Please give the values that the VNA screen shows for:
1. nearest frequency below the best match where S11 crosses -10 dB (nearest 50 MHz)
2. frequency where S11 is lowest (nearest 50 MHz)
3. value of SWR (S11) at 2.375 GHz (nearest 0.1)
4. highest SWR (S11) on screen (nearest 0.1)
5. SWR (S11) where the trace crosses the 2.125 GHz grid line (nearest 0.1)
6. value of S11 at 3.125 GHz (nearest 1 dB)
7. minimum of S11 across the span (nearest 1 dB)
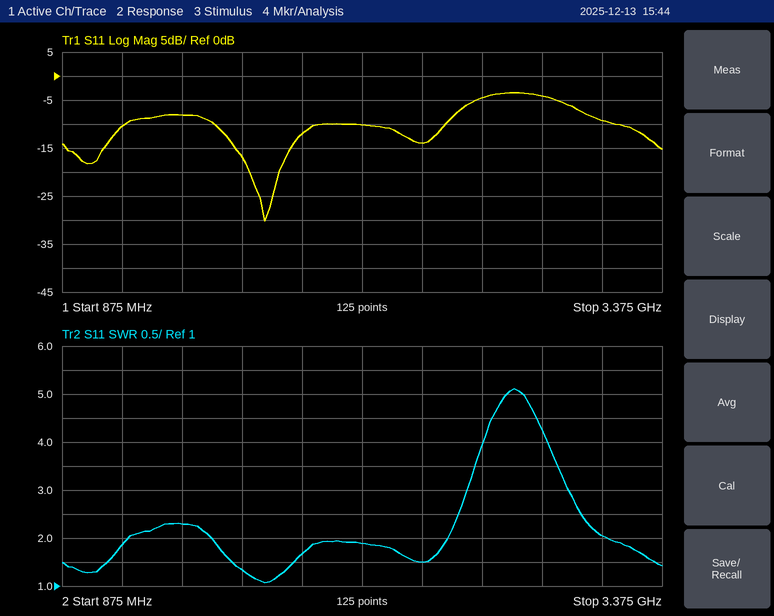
1.50 GHz
1.70 GHz
1.5
5.1
1.9
-9 dB
-30 dB
